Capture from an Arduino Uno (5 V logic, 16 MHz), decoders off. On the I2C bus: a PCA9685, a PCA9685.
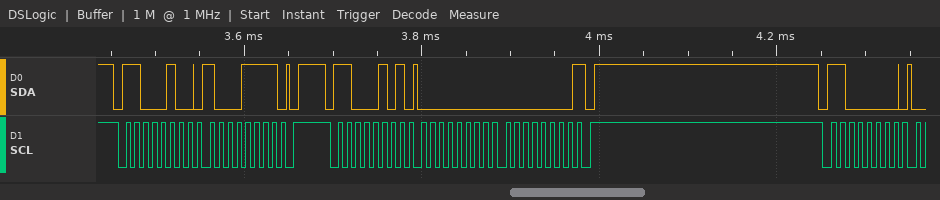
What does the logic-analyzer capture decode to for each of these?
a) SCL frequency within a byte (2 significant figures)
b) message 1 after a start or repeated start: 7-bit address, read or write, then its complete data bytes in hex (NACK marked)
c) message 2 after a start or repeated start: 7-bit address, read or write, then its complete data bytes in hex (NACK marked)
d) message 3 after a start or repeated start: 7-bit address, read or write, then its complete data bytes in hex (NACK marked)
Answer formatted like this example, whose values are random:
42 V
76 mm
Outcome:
100 kHz
0x62 write: 8F
0x62 read: 00 00 NACK
0x60 write
